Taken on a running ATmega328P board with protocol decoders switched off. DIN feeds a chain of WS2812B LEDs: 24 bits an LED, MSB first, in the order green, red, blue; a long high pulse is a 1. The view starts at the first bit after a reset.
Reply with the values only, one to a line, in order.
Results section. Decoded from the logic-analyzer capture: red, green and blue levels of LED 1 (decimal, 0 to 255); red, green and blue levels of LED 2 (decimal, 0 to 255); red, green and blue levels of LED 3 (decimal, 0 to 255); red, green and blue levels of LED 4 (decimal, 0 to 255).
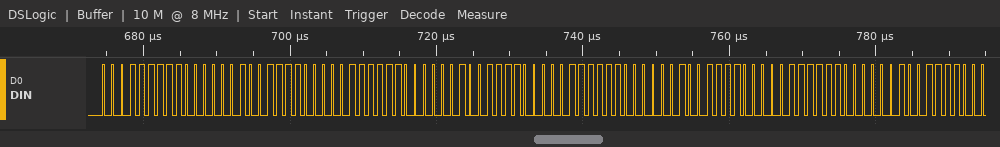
129, 31, 60
129, 31, 60
129, 31, 60
129, 31, 60
